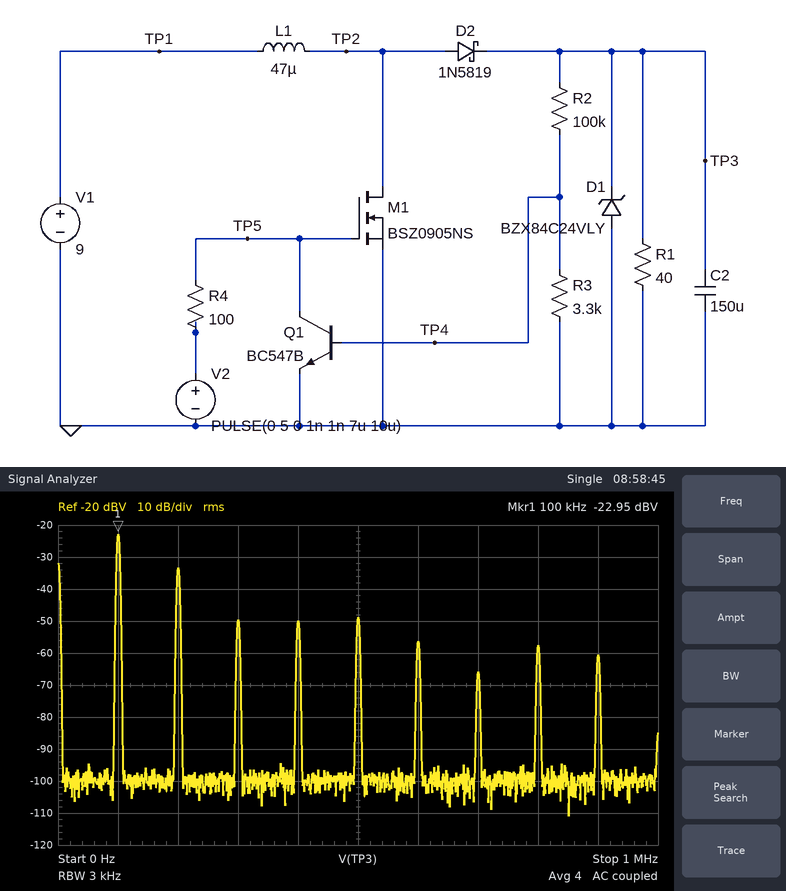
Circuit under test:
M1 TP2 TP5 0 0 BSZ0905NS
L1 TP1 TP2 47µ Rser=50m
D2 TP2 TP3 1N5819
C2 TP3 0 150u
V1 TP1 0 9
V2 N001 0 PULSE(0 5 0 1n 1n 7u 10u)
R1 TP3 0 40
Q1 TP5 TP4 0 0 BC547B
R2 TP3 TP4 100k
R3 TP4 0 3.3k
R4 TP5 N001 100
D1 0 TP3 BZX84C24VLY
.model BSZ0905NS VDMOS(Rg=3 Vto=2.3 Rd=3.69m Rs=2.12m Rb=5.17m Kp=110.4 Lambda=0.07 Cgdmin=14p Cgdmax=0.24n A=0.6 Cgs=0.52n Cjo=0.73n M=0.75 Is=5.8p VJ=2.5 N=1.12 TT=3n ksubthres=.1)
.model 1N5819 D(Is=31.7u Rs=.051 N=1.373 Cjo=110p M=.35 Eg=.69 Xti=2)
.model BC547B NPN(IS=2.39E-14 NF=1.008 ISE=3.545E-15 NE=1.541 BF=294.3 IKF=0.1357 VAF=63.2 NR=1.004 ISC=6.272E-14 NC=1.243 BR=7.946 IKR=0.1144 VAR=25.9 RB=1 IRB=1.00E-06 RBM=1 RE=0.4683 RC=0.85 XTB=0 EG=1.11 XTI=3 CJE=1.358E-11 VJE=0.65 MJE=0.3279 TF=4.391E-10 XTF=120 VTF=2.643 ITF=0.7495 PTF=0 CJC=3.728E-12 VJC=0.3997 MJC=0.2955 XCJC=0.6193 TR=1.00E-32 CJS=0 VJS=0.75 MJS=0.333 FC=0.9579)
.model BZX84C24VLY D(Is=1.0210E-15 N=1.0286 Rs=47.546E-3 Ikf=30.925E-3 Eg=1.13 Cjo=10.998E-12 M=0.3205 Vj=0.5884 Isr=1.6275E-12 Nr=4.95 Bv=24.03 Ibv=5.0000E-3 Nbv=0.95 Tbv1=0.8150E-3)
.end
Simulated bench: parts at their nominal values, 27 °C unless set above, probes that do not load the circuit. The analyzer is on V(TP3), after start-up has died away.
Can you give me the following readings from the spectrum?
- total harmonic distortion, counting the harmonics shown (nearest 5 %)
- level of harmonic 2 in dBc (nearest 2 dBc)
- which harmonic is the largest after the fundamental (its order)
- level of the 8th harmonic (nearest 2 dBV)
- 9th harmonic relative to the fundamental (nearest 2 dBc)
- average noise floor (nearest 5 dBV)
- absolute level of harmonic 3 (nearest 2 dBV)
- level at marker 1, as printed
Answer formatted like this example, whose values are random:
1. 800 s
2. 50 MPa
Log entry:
1. 30 %
2. -10 dBc
3. 2
4. -58 dBV
5. -38 dBc
6. -100 dBV
7. -50 dBV
8. -22.95 dBV
